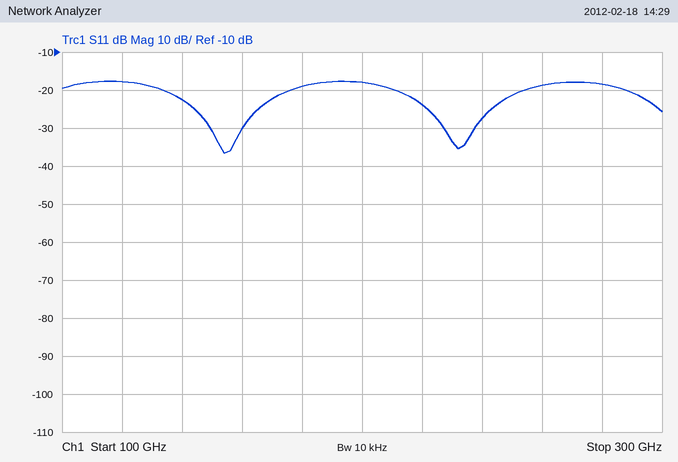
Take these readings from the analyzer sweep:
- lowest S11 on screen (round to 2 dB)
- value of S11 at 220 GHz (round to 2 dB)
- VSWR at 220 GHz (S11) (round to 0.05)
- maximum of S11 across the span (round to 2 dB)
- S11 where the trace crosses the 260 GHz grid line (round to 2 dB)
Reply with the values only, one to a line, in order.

-36 dB
-24 dB
1.15
-18 dB
-18 dB
